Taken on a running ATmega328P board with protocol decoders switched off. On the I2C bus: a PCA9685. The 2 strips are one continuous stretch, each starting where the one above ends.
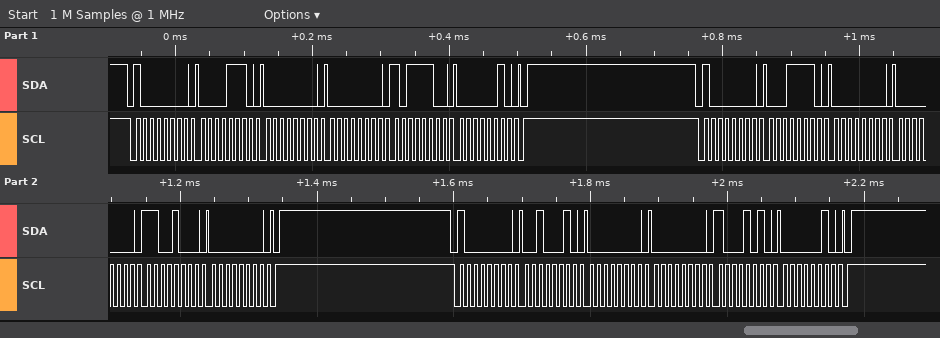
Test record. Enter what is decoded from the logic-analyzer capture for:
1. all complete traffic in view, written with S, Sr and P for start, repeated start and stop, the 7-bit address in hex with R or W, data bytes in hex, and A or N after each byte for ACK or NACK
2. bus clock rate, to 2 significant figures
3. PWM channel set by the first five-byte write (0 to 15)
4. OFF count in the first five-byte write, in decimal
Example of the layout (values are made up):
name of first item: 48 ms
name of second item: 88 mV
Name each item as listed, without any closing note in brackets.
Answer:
all complete traffic in view, written with S, Sr and P for start, repeated start and stop, the 7-bit address in hex with R or W, data bytes in hex, and A or N after each byte for ACK or NACK: S 40W A 0E A 00 A 00 A BC A 02 A P S 40W A 1E A 00 A 00 A C8 A 00 A P S 40W A 22 A 00 A 00 A 8A A 02 A P
bus clock rate, to 2 significant figures: 100 kHz
PWM channel set by the first five-byte write: 2
OFF count in the first five-byte write, in decimal: 700
